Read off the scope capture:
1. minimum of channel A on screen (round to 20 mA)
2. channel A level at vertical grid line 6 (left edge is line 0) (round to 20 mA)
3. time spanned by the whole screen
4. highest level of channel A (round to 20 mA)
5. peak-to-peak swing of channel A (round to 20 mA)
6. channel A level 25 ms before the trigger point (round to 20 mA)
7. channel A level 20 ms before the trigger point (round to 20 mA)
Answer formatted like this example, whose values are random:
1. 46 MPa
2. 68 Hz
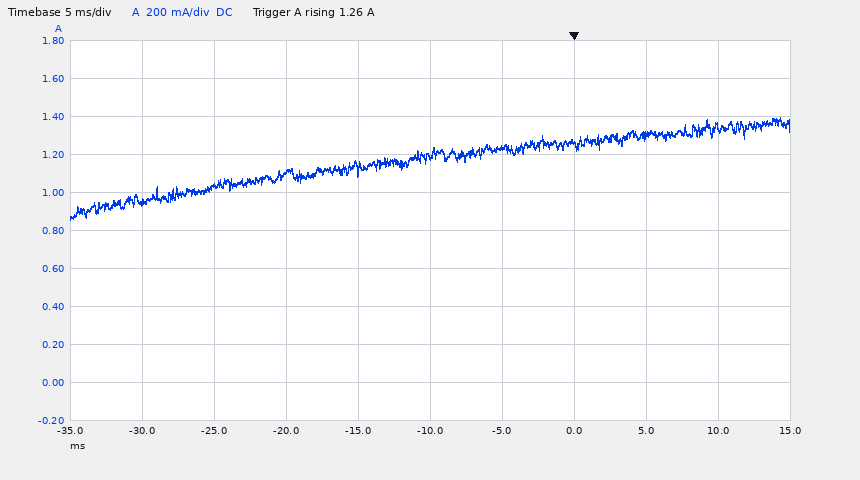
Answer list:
1. 860 mA
2. 1.24 A
3. 50 ms
4. 1.40 A
5. 540 mA
6. 1.04 A
7. 1.10 A
